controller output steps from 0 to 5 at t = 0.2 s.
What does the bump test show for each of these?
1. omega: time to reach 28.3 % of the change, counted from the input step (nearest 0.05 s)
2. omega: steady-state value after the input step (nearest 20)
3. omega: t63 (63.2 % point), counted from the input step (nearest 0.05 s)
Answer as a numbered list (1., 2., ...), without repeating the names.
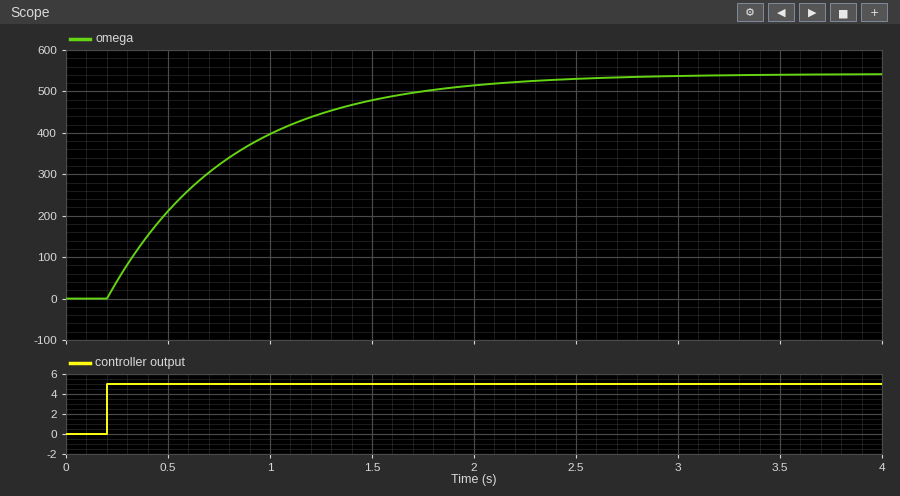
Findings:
1. 0.20 s
2. 540
3. 0.60 s
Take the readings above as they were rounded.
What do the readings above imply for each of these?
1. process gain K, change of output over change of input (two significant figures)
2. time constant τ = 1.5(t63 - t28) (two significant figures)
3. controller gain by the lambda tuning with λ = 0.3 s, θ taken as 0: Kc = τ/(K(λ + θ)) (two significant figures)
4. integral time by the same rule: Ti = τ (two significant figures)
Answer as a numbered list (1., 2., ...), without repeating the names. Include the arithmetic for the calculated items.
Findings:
1. (540 - 0) / 5 = 110
2. 1.5 × (0.6 - 0.2) = 0.60 s
3. 0.6 / (110 × (0.3 + 0)) = 0.018
4. 0.60 s
